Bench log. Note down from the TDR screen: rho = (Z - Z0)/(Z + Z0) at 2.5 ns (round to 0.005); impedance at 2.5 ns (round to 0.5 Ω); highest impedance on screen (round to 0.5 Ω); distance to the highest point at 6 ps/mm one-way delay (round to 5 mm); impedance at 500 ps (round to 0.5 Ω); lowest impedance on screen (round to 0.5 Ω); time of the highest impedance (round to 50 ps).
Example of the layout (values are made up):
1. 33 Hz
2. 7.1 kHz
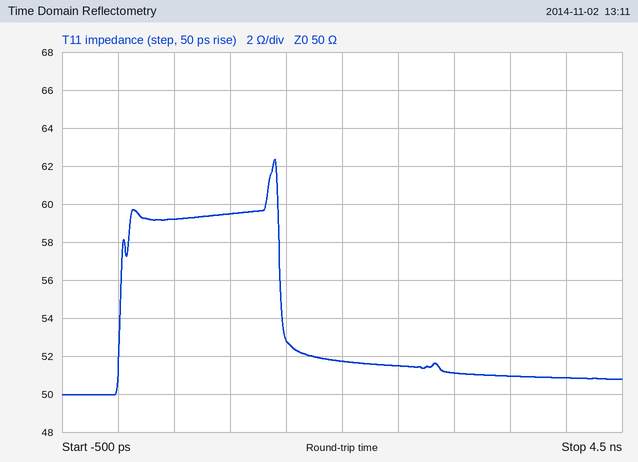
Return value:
1. +0.015
2. 51.5 Ω
3. 62.5 Ω
4. 115 mm
5. 59.0 Ω
6. 50.0 Ω
7. 1.40 ns
